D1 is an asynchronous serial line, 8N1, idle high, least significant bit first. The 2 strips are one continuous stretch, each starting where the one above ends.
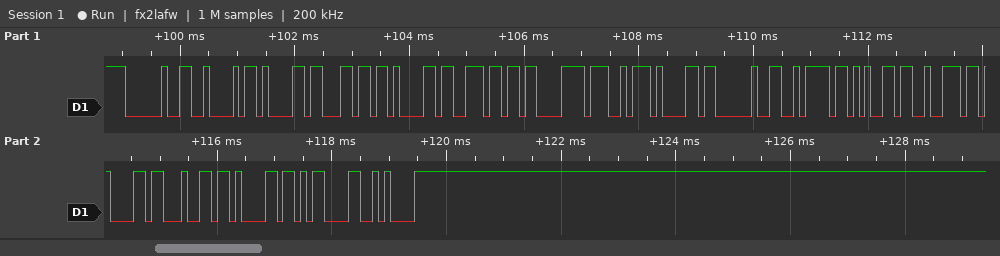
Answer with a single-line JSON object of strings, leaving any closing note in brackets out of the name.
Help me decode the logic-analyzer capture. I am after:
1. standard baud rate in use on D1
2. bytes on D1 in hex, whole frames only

{"standard baud rate in use on D1": "9600 baud", "bytes on D1 in hex, whole frames only": "0x20 0x42 0x61 0x6C 0x61 0x6E 0xC3 0xA7 0x61 0x20 0x7A 0x65 0x72 0x61 0x64 0x61 0x0D 0x0A"}
